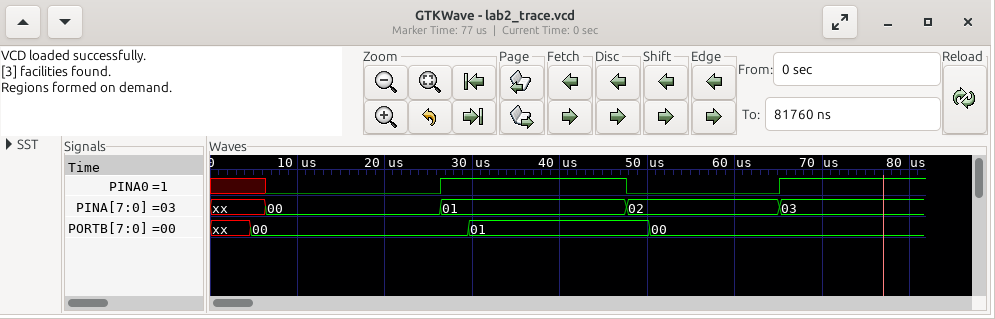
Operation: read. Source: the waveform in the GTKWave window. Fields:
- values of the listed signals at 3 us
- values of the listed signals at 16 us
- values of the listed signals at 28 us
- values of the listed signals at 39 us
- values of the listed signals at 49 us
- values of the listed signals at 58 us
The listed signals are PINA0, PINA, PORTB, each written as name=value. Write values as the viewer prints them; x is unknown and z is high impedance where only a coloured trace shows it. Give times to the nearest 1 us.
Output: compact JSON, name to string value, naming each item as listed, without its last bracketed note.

{"values of the listed signals at 3 us": "PINA0=x, PINA=xx, PORTB=xx", "values of the listed signals at 16 us": "PINA0=0, PINA=00, PORTB=00", "values of the listed signals at 28 us": "PINA0=1, PINA=01, PORTB=00", "values of the listed signals at 39 us": "PINA0=1, PINA=01, PORTB=01", "values of the listed signals at 49 us": "PINA0=0, PINA=02, PORTB=01", "values of the listed signals at 58 us": "PINA0=0, PINA=02, PORTB=00"}
